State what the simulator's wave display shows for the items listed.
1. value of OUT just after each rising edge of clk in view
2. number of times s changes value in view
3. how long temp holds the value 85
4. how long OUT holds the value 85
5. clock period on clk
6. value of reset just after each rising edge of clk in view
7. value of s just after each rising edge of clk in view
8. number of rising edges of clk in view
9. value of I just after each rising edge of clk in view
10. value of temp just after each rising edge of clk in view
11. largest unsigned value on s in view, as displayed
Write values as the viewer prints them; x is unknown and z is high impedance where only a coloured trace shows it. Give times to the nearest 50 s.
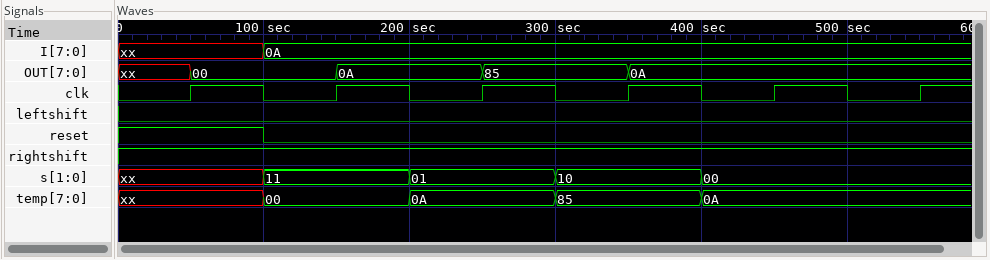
00, 0A, 85, 0A, 0A, 0A
4
100 s
100 s
100 s
1 0 0 0 0 0
xx, 11, 01, 10, 00, 00
6
xx, 0A, 0A, 0A, 0A, 0A
xx, 00, 0A, 85, 0A, 0A
11
